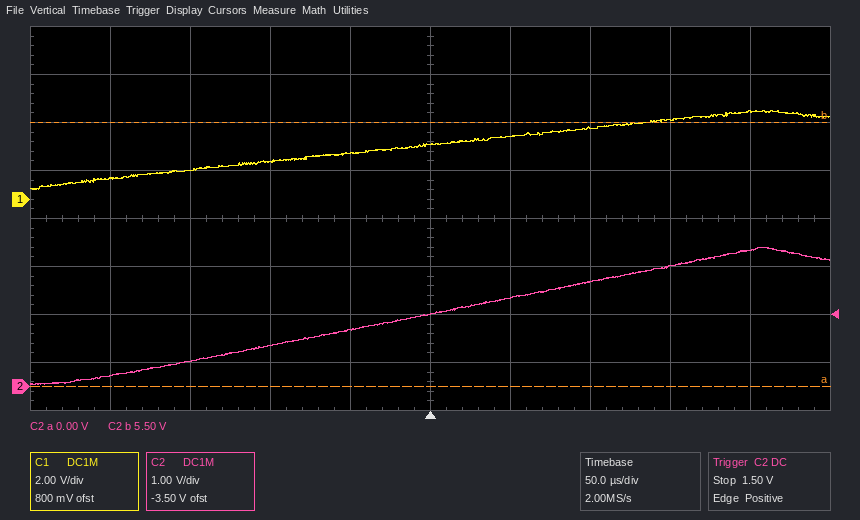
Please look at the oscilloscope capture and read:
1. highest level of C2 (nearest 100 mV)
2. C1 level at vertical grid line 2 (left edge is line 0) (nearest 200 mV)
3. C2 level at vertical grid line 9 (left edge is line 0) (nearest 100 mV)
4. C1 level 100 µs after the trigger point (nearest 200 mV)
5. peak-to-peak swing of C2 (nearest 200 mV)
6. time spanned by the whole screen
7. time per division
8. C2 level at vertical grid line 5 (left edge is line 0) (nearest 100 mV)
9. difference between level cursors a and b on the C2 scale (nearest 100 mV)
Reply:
2.9 V
1.2 V
2.8 V
3.0 V
2.8 V
500 µs
50 µs
1.5 V
5.5 V
